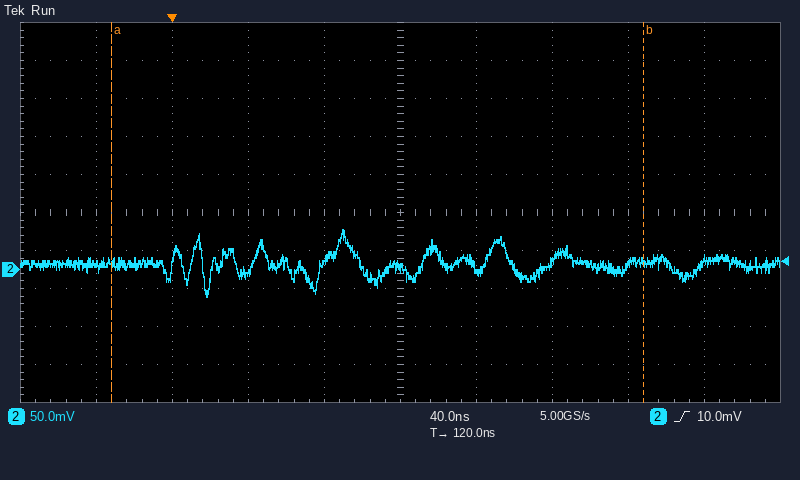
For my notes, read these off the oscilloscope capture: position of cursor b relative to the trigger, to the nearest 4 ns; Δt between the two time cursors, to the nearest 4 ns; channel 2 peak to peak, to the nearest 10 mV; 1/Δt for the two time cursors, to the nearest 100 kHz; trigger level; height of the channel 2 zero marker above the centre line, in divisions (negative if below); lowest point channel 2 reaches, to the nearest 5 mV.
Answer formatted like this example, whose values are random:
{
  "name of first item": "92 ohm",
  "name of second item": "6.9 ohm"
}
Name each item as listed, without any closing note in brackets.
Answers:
{
  "position of cursor b relative to the trigger, to the nearest 4 ns": "+248 ns",
  "Δt between the two time cursors, to the nearest 4 ns": "280 ns",
  "channel 2 peak to peak, to the nearest 10 mV": "90 mV",
  "1/Δt for the two time cursors, to the nearest 100 kHz": "3.6 MHz",
  "trigger level": "10.0 mV",
  "height of the channel 2 zero marker above the centre line, in divisions": "-1.5 div",
  "lowest point channel 2 reaches, to the nearest 5 mV": "-35 mV"
}
